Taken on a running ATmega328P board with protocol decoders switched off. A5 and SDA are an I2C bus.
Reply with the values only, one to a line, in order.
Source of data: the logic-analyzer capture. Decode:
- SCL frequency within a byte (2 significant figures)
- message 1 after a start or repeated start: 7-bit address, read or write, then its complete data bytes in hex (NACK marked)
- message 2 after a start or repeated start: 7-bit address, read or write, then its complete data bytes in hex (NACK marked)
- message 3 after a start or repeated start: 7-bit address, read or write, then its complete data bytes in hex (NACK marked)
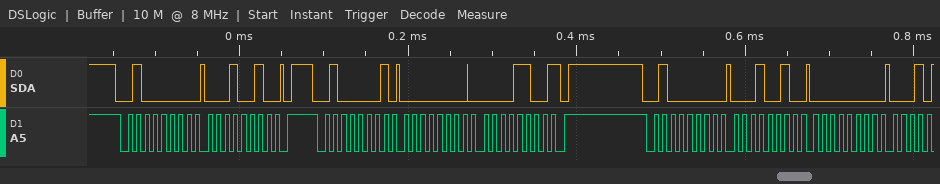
100 kHz
0x20 write: 12
0x20 read: 00 0C NACK
0x20 write: 12 00
